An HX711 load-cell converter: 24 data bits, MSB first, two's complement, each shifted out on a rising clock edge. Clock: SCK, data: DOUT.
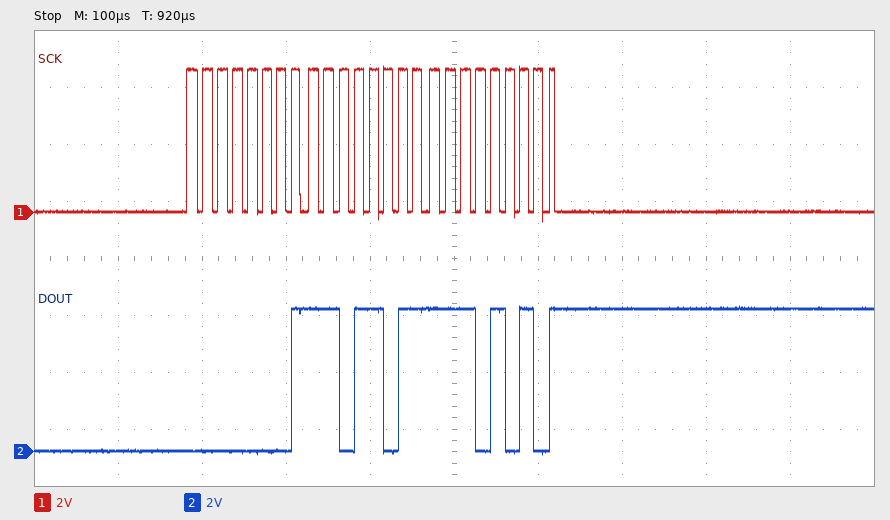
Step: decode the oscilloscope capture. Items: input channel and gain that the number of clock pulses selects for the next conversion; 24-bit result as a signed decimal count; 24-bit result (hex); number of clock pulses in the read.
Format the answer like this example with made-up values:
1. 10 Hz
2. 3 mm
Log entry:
1. channel A, gain 128
2. 121834
3. 0x01DBEA
4. 25
